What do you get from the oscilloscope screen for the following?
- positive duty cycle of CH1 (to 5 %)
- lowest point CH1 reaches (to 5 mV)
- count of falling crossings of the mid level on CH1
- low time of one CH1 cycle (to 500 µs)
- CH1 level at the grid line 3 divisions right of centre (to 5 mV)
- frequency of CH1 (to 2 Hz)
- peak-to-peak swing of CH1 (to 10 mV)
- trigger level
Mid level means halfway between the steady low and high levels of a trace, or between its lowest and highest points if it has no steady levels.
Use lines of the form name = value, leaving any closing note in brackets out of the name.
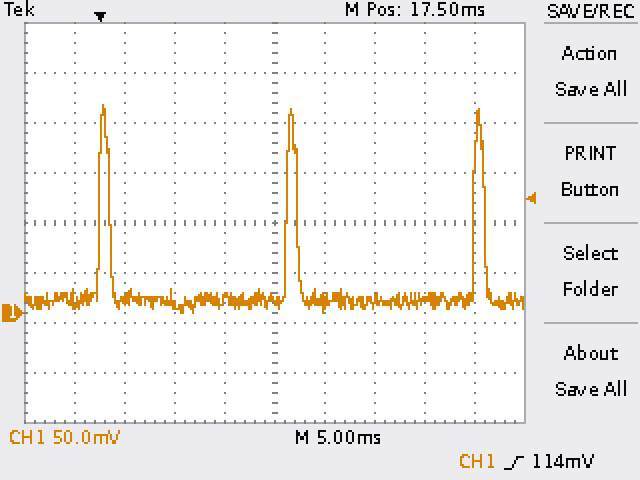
positive duty cycle of CH1 = 5 %
lowest point CH1 reaches = 0 mV
count of falling crossings of the mid level on CH1 = 3
low time of one CH1 cycle = 17.5 ms
CH1 level at the grid line 3 divisions right of centre = 10 mV
frequency of CH1 = 54 Hz
peak-to-peak swing of CH1 = 210 mV
trigger level = 114 mV
